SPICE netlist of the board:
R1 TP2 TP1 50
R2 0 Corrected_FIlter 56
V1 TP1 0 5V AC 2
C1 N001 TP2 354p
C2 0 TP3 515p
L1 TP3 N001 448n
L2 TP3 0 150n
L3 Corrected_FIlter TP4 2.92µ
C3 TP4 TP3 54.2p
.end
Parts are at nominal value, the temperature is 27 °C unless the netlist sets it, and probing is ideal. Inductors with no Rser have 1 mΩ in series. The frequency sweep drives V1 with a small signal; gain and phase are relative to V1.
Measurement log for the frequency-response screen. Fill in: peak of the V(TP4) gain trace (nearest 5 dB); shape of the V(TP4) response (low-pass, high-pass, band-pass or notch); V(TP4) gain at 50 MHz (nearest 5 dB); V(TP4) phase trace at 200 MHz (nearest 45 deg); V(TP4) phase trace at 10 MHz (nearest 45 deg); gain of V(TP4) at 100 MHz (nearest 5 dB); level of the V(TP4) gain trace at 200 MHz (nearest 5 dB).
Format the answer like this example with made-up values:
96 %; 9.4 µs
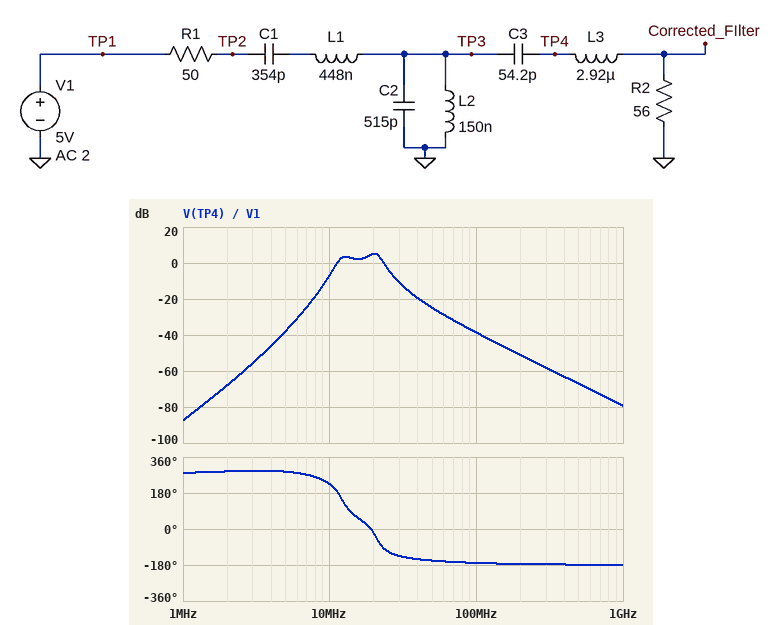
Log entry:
5 dB; band-pass; -25 dB; -180 deg; 225 deg; -40 dB; -50 dB
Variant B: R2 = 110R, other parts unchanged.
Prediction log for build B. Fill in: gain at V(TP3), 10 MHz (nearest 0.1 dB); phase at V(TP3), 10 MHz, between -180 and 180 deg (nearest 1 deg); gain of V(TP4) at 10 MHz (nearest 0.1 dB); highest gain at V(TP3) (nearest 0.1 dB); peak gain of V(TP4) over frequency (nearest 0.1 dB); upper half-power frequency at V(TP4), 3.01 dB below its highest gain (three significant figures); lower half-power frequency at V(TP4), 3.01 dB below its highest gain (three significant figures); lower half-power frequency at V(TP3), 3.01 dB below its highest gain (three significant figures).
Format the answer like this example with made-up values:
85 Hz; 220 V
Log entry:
-11.0 dB; 89 deg; -8.2 dB; 0.7 dB; 4.4 dB; 22.6 MHz; 16.5 MHz; 17.9 MHz
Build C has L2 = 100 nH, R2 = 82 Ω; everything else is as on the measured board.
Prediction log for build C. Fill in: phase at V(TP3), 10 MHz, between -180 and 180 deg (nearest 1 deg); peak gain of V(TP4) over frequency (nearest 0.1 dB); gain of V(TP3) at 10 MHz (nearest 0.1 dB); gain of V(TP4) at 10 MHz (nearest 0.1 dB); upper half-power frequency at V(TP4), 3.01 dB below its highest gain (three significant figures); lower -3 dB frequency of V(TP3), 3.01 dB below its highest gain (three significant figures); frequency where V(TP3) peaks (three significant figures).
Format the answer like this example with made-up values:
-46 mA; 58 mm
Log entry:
98 deg; 5.0 dB; -15.8 dB; -12.5 dB; 25.9 MHz; 22.6 MHz; 24.4 MHz
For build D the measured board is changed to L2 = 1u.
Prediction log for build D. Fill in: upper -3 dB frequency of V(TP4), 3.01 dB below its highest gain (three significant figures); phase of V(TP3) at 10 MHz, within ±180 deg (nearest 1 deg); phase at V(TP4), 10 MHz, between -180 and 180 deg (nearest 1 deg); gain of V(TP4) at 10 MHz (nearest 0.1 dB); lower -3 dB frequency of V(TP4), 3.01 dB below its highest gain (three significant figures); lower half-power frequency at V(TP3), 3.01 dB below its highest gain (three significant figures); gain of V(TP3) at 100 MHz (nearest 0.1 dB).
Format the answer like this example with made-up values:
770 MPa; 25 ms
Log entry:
15.6 MHz; -35 deg; 101 deg; -1.9 dB; 11.7 MHz; 4.77 MHz; -39.0 dB
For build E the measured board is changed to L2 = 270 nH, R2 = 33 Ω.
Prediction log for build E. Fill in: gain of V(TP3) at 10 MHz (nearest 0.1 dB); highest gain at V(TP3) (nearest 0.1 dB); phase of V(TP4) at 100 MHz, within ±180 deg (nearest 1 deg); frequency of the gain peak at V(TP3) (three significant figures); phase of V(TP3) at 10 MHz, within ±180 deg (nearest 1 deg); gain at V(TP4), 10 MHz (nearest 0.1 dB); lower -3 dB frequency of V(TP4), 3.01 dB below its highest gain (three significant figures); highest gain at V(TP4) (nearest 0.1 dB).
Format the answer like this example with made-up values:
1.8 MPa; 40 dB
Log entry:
-2.0 dB; -0.5 dB; -170 deg; 16.6 MHz; 49 deg; 2.2 dB; 10.8 MHz; 9.0 dB
